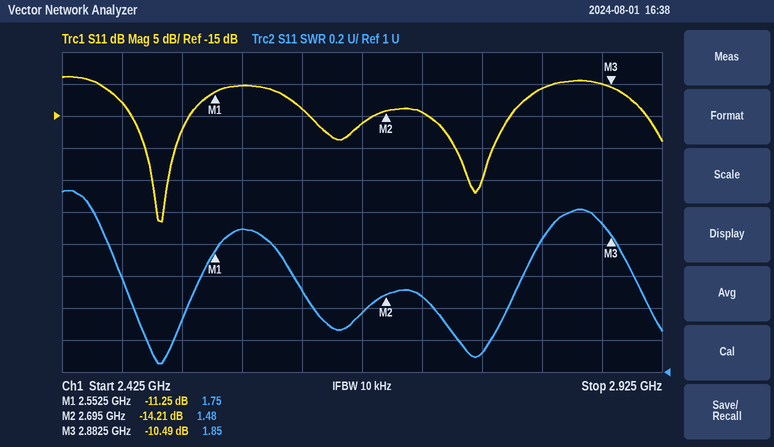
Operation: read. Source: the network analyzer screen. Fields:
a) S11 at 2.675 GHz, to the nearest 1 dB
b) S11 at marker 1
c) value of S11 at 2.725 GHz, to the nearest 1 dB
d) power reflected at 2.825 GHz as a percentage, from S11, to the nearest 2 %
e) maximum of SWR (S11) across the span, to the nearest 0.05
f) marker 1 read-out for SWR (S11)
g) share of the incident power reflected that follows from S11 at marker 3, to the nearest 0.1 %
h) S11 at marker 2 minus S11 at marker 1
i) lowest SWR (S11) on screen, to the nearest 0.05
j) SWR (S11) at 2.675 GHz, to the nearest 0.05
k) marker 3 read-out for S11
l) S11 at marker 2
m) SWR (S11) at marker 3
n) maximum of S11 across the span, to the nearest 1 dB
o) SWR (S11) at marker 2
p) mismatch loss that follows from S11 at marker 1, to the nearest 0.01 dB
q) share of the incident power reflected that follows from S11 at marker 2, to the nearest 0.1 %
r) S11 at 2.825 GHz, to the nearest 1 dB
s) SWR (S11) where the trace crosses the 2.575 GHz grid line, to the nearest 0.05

-16 dB
-11.25 dB
-14 dB
8 %
2.15
1.75
8.9 %
-2.96 dB
1.05
1.35
-10.49 dB
-14.21 dB
1.85
-9 dB
1.48
0.34 dB
3.8 %
-11 dB
1.90
